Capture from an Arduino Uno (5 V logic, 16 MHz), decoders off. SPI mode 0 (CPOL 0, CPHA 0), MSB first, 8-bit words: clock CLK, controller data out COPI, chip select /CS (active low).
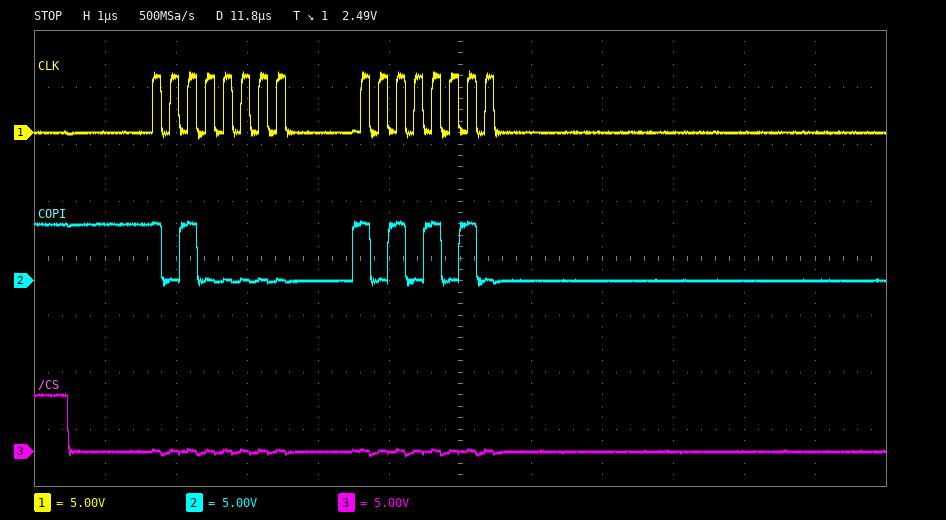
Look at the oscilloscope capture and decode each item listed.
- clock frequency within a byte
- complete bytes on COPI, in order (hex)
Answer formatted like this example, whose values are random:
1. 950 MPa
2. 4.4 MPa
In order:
1. 4 MHz
2. A0 AA
